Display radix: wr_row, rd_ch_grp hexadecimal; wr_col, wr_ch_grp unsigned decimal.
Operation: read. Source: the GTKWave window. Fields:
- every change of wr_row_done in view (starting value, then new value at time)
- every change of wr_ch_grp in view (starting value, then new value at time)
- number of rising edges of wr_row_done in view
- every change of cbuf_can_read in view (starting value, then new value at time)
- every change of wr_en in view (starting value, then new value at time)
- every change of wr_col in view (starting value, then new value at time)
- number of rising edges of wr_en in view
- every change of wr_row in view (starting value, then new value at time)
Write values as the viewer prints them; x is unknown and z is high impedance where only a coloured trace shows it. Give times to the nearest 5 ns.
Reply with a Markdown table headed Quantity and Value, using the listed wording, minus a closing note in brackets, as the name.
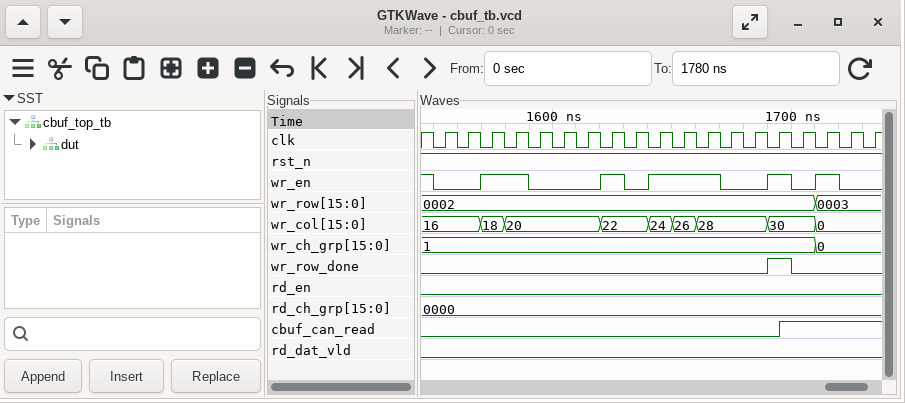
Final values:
| Quantity | Value |
|---|---|
| every change of wr_row_done in view | 0, 1 at 1690 ns, 0 at 1700 ns |
| every change of wr_ch_grp in view | 1, 0 at 1710 ns |
| number of rising edges of wr_row_done in view | 1 |
| every change of cbuf_can_read in view | 0, 1 at 1695 ns |
| every change of wr_en in view | 1, 0 at 1550 ns, 1 at 1570 ns, 0 at 1590 ns, 1 at 1620 ns, 0 at 1630 ns, 1 at 1640 ns, 0 at 1670 ns, 1 at 1690 ns, 0 at 1700 ns, 1 at 1710 ns, 0 at 1720 ns |
| every change of wr_col in view | 16, 18 at 1570 ns, 20 at 1580 ns, 22 at 1620 ns, 24 at 1640 ns, 26 at 1650 ns, 28 at 1660 ns, 30 at 1690 ns, 0 at 1710 ns |
| number of rising edges of wr_en in view | 5 |
| every change of wr_row in view | 0002, 0003 at 1710 ns |
